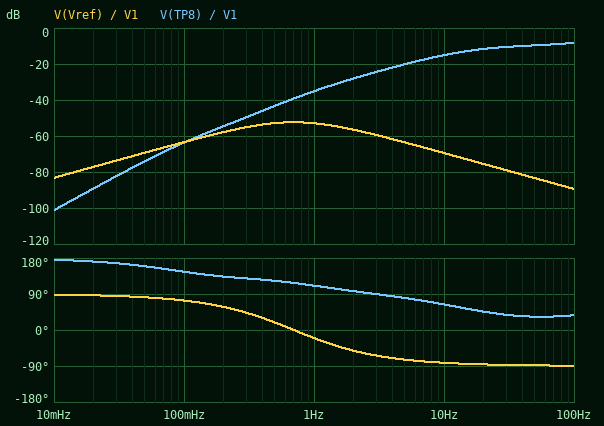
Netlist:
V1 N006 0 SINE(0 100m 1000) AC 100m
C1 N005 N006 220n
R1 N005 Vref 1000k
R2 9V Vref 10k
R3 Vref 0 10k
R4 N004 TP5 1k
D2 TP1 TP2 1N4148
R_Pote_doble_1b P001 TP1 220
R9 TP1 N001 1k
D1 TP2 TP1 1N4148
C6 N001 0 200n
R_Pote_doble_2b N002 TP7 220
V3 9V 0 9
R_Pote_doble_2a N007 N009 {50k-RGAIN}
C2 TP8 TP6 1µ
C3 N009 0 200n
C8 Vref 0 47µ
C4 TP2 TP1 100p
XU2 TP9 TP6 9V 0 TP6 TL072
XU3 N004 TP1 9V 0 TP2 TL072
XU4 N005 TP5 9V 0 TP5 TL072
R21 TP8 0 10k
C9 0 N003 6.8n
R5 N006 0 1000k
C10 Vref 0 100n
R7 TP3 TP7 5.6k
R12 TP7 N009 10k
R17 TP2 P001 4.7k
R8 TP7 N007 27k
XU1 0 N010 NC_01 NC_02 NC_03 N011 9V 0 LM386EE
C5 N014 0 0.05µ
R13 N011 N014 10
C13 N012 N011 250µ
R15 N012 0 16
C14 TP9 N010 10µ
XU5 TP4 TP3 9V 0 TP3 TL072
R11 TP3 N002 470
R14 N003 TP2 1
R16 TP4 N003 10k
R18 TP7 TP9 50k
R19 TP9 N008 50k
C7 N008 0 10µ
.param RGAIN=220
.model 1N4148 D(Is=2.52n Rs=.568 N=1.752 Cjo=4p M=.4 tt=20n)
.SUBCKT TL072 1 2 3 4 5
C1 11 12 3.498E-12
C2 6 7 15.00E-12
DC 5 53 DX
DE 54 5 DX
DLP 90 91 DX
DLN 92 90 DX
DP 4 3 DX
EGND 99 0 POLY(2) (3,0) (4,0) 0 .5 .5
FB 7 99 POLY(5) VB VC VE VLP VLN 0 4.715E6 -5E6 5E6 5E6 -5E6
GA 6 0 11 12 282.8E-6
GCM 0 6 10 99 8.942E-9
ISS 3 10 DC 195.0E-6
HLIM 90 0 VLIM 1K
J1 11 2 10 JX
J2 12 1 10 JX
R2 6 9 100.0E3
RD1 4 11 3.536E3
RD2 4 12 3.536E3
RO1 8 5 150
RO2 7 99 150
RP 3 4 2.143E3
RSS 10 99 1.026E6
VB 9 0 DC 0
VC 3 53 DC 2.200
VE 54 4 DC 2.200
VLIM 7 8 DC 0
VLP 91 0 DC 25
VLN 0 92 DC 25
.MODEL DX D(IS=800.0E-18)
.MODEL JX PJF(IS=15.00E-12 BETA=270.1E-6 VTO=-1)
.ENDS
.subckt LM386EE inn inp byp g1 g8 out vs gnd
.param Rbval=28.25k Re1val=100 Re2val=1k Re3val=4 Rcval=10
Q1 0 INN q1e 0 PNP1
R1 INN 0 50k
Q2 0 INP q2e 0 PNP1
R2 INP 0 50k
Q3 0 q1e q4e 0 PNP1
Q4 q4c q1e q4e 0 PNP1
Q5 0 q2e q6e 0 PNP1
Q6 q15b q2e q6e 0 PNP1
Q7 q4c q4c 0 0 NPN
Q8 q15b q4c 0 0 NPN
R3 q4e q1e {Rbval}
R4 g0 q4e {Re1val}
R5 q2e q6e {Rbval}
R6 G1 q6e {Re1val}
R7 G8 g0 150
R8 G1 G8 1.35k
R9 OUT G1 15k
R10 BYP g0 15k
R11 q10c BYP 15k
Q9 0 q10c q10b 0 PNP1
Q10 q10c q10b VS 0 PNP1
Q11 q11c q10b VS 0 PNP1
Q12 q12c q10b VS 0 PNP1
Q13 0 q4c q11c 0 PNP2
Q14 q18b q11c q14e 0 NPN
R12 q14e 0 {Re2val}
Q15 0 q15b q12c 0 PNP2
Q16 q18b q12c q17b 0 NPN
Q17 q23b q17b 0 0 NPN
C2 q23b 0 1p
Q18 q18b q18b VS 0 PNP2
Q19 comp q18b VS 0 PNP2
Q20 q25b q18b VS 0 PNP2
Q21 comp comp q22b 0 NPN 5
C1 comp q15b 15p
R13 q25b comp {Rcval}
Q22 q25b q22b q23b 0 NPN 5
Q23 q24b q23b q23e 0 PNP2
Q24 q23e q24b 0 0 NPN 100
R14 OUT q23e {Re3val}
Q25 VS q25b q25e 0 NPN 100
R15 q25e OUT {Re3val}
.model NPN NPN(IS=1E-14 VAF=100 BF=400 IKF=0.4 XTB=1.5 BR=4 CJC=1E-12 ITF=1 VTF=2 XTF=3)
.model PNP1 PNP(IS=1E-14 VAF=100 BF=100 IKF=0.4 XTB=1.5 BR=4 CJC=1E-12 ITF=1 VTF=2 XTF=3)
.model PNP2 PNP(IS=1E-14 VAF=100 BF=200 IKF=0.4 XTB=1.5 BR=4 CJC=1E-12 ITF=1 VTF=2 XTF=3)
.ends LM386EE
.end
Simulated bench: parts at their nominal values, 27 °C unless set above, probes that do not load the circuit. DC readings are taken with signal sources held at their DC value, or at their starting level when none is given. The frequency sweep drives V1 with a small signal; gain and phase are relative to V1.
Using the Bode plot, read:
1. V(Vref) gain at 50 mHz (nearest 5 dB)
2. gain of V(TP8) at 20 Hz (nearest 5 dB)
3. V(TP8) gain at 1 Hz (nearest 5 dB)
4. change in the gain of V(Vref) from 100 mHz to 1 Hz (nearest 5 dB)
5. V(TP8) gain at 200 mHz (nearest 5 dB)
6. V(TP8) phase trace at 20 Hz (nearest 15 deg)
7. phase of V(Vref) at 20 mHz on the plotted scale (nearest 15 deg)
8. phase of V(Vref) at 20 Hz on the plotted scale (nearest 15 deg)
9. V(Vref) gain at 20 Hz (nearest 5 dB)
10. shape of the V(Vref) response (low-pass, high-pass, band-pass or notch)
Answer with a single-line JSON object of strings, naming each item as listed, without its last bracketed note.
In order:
{"V(Vref) gain at 50 mHz": "-70 dB", "gain of V(TP8) at 20 Hz": "-10 dB", "V(TP8) gain at 1 Hz": "-35 dB", "change in the gain of V(Vref) from 100 mHz to 1 Hz": "10 dB", "V(TP8) gain at 200 mHz": "-55 dB", "V(TP8) phase trace at 20 Hz": "45 deg", "phase of V(Vref) at 20 mHz on the plotted scale": "90 deg", "phase of V(Vref) at 20 Hz on the plotted scale": "-90 deg", "V(Vref) gain at 20 Hz": "-75 dB", "shape of the V(Vref) response": "band-pass"}
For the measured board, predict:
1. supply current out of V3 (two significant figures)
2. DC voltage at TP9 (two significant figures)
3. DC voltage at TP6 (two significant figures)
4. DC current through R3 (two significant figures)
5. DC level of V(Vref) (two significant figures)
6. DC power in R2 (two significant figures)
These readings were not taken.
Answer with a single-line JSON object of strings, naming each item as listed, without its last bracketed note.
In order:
{"supply current out of V3": "22 mA", "DC voltage at TP9": "4.5 V", "DC voltage at TP6": "4.5 V", "DC current through R3": "450 µA", "DC level of V(Vref)": "4.5 V", "DC power in R2": "2.0 mW"}
